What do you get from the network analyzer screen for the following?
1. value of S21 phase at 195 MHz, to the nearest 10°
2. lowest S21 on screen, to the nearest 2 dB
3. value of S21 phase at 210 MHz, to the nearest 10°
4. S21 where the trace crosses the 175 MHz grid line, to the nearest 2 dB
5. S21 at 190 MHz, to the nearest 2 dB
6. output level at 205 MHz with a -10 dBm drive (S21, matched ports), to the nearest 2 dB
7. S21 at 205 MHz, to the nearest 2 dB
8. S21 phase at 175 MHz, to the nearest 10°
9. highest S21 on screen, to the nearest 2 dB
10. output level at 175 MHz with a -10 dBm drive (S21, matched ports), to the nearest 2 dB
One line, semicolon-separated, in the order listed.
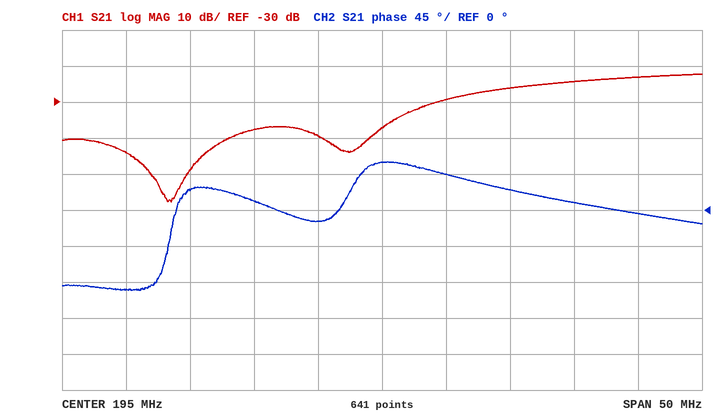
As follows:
60°; -58 dB; 10°; -44 dB; -40 dB; -36 dBm; -26 dB; -100°; -22 dB; -54 dBm
